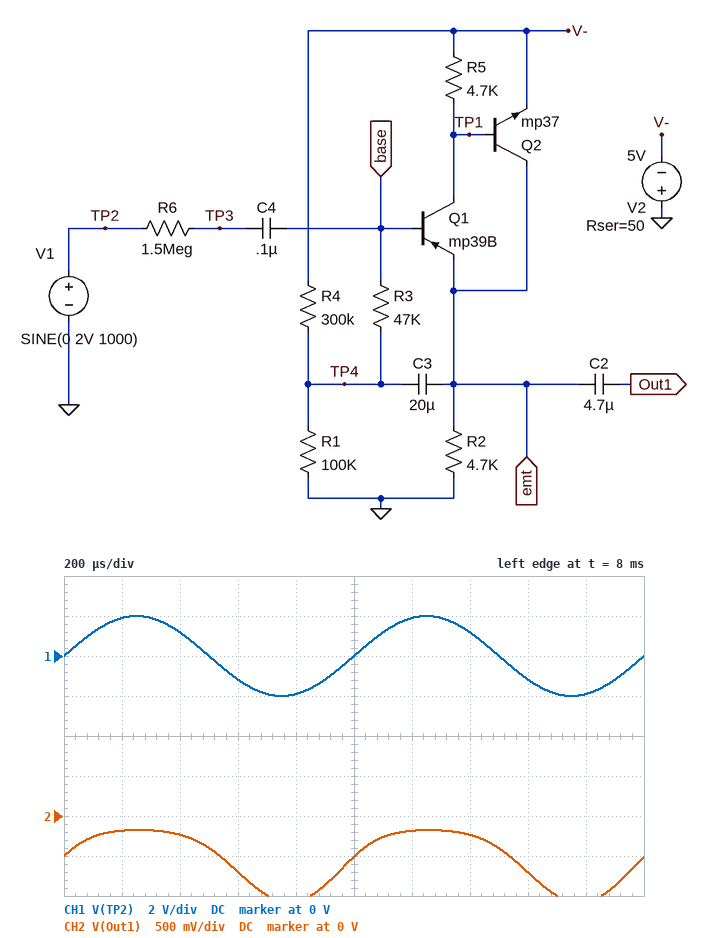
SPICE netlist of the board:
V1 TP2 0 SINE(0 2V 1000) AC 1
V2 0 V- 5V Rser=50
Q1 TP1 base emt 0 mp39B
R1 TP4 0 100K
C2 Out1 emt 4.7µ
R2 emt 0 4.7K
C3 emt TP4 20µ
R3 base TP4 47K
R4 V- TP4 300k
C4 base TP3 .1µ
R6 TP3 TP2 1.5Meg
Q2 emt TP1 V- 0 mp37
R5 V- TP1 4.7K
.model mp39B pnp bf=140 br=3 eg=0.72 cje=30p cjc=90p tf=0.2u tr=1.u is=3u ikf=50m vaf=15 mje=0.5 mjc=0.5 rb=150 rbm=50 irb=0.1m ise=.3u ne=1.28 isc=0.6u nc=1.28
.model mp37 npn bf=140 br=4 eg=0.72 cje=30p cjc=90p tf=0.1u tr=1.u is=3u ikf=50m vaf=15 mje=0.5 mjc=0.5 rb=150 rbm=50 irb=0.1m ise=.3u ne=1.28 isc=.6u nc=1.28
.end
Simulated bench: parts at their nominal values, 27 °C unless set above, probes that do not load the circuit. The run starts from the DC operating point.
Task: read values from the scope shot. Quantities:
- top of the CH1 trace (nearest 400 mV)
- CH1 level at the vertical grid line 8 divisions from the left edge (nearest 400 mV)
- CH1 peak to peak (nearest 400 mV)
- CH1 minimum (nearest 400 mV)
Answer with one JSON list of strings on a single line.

["2.0 V", "-1.2 V", "4.0 V", "-2.0 V"]
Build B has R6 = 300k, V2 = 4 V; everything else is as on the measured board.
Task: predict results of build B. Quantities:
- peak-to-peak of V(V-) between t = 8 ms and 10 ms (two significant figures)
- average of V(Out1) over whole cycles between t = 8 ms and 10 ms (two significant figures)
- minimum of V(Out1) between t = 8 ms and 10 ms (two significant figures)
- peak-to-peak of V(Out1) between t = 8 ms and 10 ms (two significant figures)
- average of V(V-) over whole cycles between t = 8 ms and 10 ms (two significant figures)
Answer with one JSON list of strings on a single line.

["18 mV", "-620 mV", "-1.7 V", "1.6 V", "-4.0 V"]
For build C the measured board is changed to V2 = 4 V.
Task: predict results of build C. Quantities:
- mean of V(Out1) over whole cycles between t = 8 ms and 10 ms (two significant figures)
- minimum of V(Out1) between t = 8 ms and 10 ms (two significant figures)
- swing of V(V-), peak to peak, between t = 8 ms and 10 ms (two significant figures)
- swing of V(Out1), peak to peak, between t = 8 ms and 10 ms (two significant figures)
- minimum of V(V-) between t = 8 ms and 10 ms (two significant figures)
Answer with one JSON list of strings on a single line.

["-480 mV", "-980 mV", "9.1 mV", "820 mV", "-4.0 V"]
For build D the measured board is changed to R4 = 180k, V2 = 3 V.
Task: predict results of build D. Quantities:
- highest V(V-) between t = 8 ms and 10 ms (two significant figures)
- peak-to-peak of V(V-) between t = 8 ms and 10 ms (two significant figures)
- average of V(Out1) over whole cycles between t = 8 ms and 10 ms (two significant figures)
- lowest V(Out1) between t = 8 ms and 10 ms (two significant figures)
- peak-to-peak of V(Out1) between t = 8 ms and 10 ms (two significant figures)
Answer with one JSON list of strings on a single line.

["-3.0 V", "8.3 mV", "-460 mV", "-910 mV", "750 mV"]
